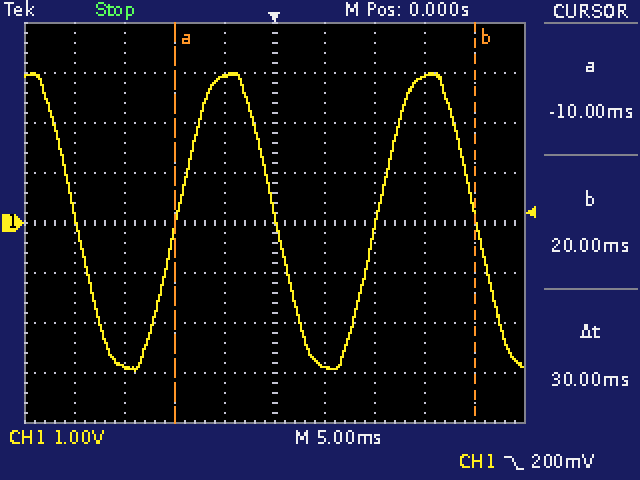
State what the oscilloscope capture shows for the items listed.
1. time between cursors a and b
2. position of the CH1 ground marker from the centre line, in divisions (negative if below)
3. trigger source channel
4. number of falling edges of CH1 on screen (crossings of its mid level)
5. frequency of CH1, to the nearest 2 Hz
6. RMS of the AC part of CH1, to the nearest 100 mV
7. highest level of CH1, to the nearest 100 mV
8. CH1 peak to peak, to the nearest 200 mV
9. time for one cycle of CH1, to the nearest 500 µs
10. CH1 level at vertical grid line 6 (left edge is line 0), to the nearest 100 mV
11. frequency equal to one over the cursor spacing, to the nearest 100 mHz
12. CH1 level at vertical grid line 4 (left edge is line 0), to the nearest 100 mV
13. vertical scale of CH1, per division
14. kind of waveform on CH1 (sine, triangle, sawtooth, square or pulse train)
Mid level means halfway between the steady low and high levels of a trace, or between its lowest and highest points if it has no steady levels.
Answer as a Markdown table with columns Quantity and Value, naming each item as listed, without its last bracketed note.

| Quantity | Value |
|---|---|
| time between cursors a and b | 30 ms |
| position of the CH1 ground marker from the centre line, in divisions | 0.0 div |
| trigger source channel | CH1 |
| number of falling edges of CH1 on screen | 3 |
| frequency of CH1, to the nearest 2 Hz | 50 Hz |
| RMS of the AC part of CH1, to the nearest 100 mV | 2.1 V |
| highest level of CH1, to the nearest 100 mV | 3.0 V |
| CH1 peak to peak, to the nearest 200 mV | 6.0 V |
| time for one cycle of CH1, to the nearest 500 µs | 20.0 ms |
| CH1 level at vertical grid line 6 (left edge is line 0), to the nearest 100 mV | -2.9 V |
| frequency equal to one over the cursor spacing, to the nearest 100 mHz | 33.3 Hz |
| CH1 level at vertical grid line 4 (left edge is line 0), to the nearest 100 mV | 2.9 V |
| vertical scale of CH1, per division | 1 V |
| kind of waveform on CH1 | sine |
